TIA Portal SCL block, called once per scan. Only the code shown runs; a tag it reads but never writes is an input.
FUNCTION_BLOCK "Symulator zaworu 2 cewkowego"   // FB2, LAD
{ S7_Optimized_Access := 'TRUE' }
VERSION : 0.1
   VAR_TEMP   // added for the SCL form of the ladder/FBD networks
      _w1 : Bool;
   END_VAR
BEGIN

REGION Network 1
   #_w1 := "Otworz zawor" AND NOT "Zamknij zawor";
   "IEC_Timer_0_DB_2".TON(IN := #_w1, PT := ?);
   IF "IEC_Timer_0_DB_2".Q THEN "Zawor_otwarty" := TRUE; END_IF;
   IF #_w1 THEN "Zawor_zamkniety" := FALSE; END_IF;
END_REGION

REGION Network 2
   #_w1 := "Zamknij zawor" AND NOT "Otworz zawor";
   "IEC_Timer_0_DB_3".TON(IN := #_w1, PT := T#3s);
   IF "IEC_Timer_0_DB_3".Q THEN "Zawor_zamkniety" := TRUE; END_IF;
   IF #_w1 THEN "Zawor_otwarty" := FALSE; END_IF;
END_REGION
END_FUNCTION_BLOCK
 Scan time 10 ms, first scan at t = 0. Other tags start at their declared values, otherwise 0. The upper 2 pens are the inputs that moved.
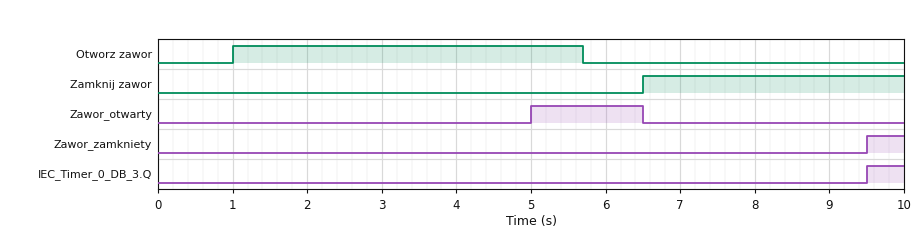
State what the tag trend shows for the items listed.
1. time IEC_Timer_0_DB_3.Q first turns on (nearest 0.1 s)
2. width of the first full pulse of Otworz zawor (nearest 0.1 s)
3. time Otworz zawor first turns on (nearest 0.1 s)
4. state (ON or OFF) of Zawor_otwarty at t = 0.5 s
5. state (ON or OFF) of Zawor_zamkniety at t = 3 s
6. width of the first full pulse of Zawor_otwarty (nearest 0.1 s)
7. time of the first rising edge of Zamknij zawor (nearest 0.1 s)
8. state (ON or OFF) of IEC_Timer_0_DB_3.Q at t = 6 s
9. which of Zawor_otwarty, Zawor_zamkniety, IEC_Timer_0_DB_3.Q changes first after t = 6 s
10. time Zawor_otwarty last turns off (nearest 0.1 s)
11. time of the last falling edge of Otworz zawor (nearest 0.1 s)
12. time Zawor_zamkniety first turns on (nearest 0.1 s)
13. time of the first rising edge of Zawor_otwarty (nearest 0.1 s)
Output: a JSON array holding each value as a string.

["9.5 s", "4.7 s", "1.0 s", "OFF", "OFF", "1.5 s", "6.5 s", "OFF", "Zawor_otwarty", "6.5 s", "5.7 s", "9.5 s", "5.0 s"]
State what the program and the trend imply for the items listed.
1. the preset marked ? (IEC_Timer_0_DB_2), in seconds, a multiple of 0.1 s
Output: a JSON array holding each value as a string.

["4.0 s"]
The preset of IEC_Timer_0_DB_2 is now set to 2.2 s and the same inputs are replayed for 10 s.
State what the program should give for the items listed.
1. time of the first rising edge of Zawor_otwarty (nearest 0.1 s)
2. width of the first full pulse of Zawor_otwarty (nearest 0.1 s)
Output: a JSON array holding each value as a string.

["3.2 s", "3.3 s"]
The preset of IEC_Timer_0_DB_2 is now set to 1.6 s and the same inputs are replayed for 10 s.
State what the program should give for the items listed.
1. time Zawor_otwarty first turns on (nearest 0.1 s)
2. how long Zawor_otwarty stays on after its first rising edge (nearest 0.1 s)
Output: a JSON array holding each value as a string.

["2.6 s", "3.9 s"]
